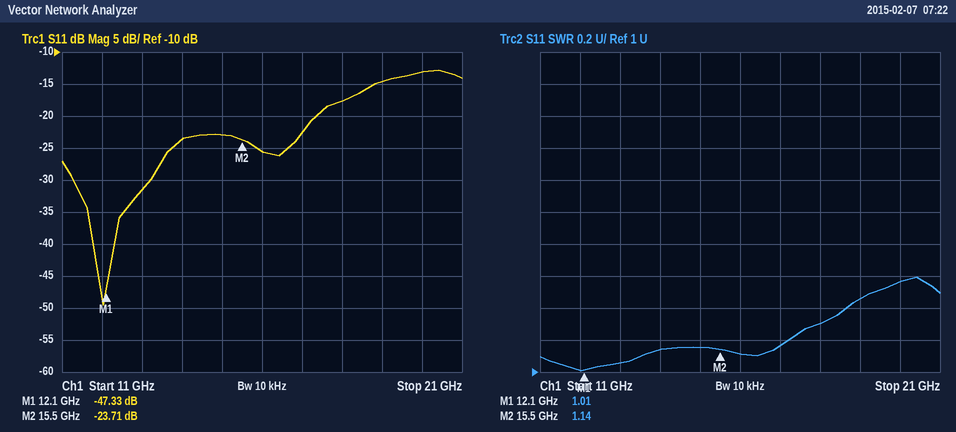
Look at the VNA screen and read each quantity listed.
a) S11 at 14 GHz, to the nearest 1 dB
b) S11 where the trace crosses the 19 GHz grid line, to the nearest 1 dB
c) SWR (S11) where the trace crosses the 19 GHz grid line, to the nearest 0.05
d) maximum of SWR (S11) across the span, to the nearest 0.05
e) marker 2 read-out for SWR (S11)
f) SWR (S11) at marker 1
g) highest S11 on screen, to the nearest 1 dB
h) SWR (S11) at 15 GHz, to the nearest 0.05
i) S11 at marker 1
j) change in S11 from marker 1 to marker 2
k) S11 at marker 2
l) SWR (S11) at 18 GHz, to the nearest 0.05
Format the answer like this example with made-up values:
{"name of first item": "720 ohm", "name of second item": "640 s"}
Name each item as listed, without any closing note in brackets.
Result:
{"S11 at 14 GHz, to the nearest 1 dB": "-24 dB", "S11 where the trace crosses the 19 GHz grid line, to the nearest 1 dB": "-15 dB", "SWR (S11) where the trace crosses the 19 GHz grid line, to the nearest 0.05": "1.45", "maximum of SWR (S11) across the span, to the nearest 0.05": "1.60", "marker 2 read-out for SWR": "1.14", "SWR (S11) at marker 1": "1.01", "highest S11 on screen, to the nearest 1 dB": "-13 dB", "SWR (S11) at 15 GHz, to the nearest 0.05": "1.15", "S11 at marker 1": "-47.33 dB", "change in S11 from marker 1 to marker 2": "23.62 dB", "S11 at marker 2": "-23.71 dB", "SWR (S11) at 18 GHz, to the nearest 0.05": "1.30"}
